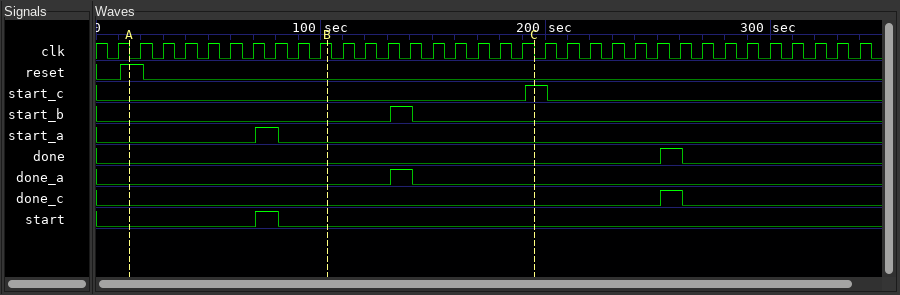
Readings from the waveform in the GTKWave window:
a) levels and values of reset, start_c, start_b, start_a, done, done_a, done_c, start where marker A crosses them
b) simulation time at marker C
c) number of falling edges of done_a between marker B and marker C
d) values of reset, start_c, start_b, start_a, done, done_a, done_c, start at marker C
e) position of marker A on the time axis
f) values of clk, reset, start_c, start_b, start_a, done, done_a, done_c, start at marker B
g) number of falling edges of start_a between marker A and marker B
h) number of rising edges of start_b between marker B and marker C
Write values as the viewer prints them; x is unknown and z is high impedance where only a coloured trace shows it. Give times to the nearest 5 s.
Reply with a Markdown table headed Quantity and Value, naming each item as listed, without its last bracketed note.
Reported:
| Quantity | Value |
|---|---|
| levels and values of reset, start_c, start_b, start_a, done, done_a, done_c, start where marker A crosses them | reset=1, start_c=0, start_b=0, start_a=0, done=0, done_a=0, done_c=0, start=0 |
| simulation time at marker C | 195 s |
| number of falling edges of done_a between marker B and marker C | 1 |
| values of reset, start_c, start_b, start_a, done, done_a, done_c, start at marker C | reset=0, start_c=1, start_b=0, start_a=0, done=0, done_a=0, done_c=0, start=0 |
| position of marker A on the time axis | 15 s |
| values of clk, reset, start_c, start_b, start_a, done, done_a, done_c, start at marker B | clk=1, reset=0, start_c=0, start_b=0, start_a=0, done=0, done_a=0, done_c=0, start=0 |
| number of falling edges of start_a between marker A and marker B | 1 |
| number of rising edges of start_b between marker B and marker C | 1 |
